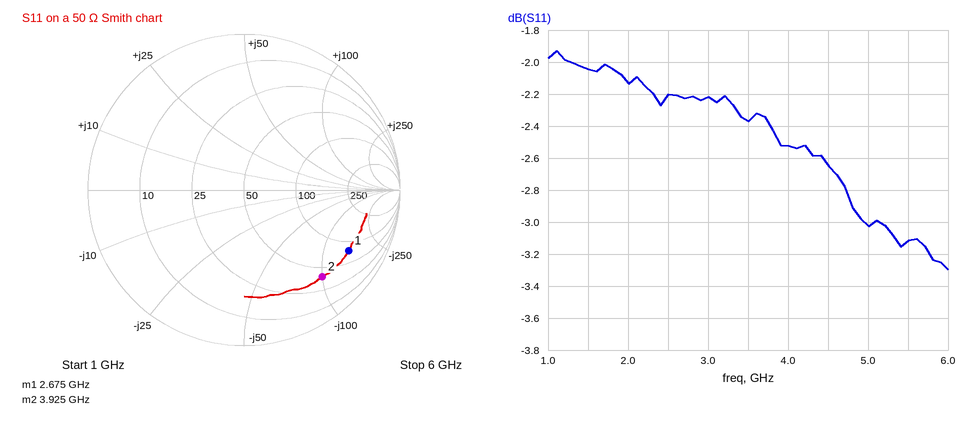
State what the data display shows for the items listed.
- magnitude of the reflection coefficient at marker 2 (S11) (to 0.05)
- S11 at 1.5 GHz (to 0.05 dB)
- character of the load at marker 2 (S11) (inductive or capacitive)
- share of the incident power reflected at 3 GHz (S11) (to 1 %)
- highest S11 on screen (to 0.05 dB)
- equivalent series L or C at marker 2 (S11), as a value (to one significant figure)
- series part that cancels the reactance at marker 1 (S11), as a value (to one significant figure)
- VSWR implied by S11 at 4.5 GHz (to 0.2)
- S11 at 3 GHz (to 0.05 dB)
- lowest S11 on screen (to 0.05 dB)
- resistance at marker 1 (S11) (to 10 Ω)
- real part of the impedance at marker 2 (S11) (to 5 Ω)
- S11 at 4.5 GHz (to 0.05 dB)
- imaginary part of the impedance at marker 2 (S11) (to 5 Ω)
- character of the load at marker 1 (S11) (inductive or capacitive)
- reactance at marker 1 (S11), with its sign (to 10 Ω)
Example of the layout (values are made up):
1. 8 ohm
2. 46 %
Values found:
1. 0.75
2. -2.05 dB
3. capacitive
4. 60 %
5. -1.95 dB
6. 400 fF
7. 9 nH
8. 6.6
9. -2.20 dB
10. -3.30 dB
11. 80 Ω
12. 40 Ω
13. -2.65 dB
14. -100 Ω
15. capacitive
16. -150 Ω
